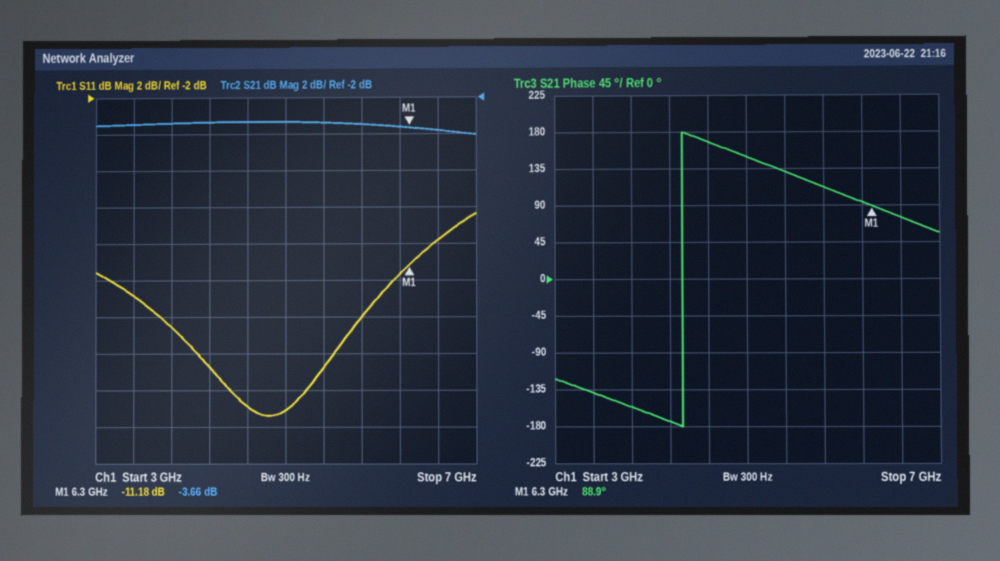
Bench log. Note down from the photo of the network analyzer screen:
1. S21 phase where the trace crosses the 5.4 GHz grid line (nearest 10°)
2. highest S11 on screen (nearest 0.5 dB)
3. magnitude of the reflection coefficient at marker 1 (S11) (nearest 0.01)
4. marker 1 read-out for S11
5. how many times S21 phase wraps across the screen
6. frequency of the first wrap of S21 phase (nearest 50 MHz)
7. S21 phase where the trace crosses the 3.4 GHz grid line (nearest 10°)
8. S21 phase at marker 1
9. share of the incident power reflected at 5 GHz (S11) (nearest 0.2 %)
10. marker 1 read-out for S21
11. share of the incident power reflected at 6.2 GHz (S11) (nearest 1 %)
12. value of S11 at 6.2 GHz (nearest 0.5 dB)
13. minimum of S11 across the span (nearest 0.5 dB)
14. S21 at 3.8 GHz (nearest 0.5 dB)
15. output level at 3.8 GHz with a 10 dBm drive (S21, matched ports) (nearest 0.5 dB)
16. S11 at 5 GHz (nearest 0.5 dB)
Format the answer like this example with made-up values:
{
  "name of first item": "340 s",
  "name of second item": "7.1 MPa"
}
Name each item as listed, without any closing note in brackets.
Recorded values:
{
  "S21 phase where the trace crosses the 5.4 GHz grid line": "130°",
  "highest S11 on screen": "-8.5 dB",
  "magnitude of the reflection coefficient at marker 1 (S11)": "0.28",
  "marker 1 read-out for S11": "-11.18 dB",
  "how many times S21 phase wraps across the screen": "1",
  "frequency of the first wrap of S21 phase": "4.35 GHz",
  "S21 phase where the trace crosses the 3.4 GHz grid line": "-140°",
  "S21 phase at marker 1": "88.9°",
  "share of the incident power reflected at 5 GHz (S11)": "1.2 %",
  "marker 1 read-out for S21": "-3.66 dB",
  "share of the incident power reflected at 6.2 GHz (S11)": "7 %",
  "value of S11 at 6.2 GHz": "-11.5 dB",
  "minimum of S11 across the span": "-19.5 dB",
  "S21 at 3.8 GHz": "-3.5 dB",
  "output level at 3.8 GHz with a 10 dBm drive (S21, matched ports)": "6.5 dBm",
  "S11 at 5 GHz": "-19.0 dB"
}
